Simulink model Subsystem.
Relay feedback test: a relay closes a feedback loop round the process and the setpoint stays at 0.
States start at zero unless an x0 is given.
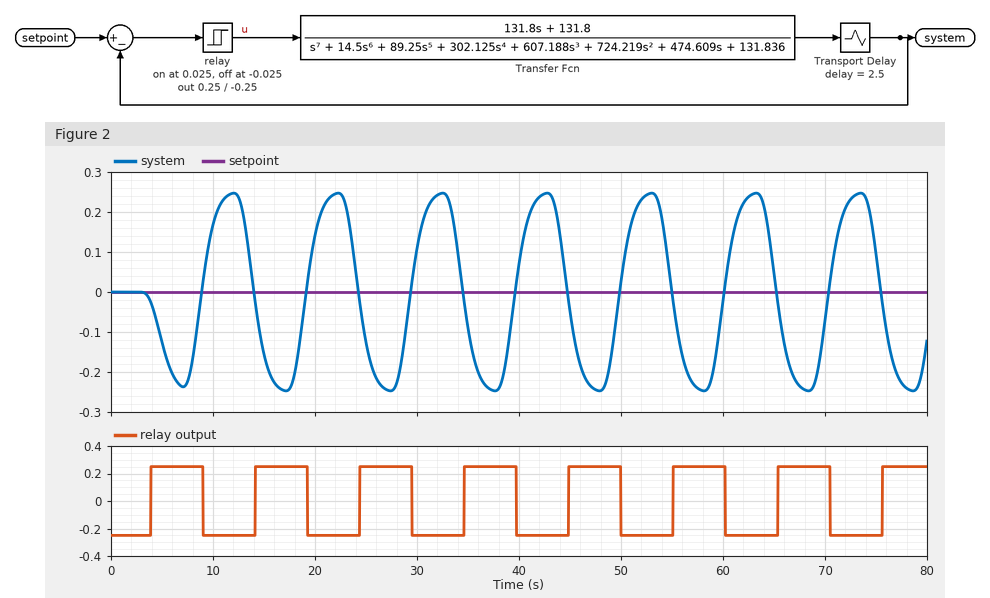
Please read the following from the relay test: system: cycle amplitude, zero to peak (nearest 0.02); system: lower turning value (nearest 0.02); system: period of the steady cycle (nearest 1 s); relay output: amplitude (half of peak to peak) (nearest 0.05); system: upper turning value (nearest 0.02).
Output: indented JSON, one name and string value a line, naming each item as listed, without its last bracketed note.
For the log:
{
  "system: cycle amplitude, zero to peak": "0.24",
  "system: lower turning value": "-0.24",
  "system: period of the steady cycle": "10 s",
  "relay output: amplitude (half of peak to peak)": "0.25",
  "system: upper turning value": "0.24"
}
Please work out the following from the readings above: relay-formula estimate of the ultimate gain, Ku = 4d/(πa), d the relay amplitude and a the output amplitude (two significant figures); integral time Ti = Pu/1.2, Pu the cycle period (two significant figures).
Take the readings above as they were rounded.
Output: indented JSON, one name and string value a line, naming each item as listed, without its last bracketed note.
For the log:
{
  "relay-formula estimate of the ultimate gain, Ku = 4d/(πa), d the relay amplitude and a the output amplitude": "1.3",
  "integral time Ti = Pu/1.2, Pu the cycle period": "8.3 s"
}
